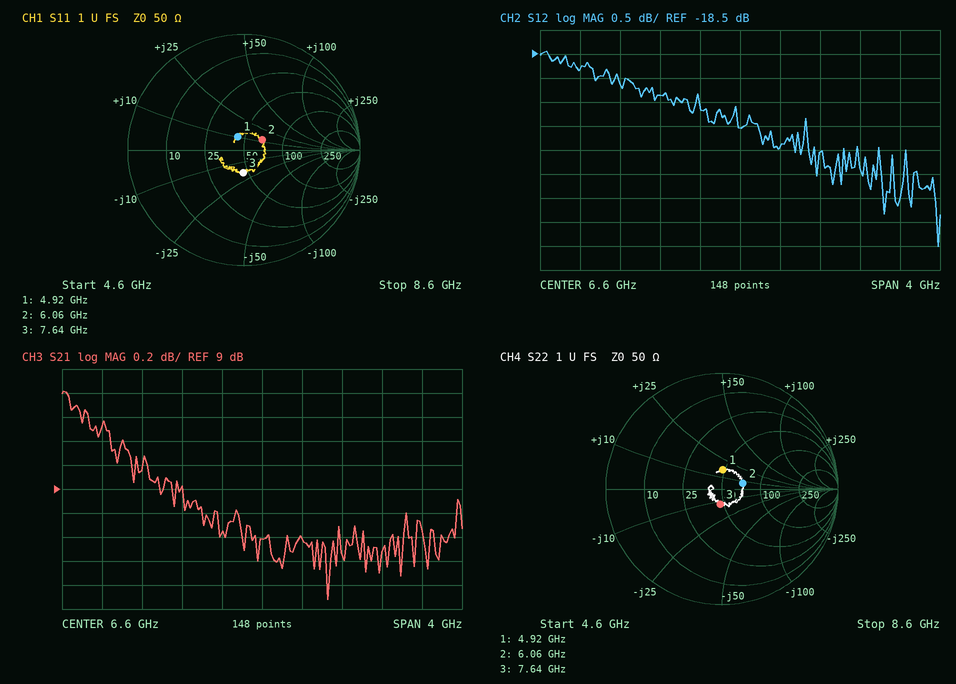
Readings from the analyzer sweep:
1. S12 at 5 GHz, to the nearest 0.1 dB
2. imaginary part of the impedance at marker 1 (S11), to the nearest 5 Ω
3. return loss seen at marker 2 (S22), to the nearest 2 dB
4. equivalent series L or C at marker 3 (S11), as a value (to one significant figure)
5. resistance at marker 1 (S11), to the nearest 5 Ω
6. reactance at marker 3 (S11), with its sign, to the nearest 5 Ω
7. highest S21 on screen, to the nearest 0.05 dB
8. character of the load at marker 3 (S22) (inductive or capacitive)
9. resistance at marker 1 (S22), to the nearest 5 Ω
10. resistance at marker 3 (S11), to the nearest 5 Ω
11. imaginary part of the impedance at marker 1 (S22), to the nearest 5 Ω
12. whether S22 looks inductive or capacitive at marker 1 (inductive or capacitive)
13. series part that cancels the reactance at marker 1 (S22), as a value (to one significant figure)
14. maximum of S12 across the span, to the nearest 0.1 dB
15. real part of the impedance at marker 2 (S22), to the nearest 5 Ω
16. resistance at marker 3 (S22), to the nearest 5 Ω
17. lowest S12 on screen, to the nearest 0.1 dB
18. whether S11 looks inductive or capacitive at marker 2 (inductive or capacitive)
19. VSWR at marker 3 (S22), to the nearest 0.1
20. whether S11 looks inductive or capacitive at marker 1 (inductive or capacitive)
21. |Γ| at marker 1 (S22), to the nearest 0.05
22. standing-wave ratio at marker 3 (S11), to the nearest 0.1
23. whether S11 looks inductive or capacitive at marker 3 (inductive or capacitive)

-18.8 dB
+10 Ω
14 dB
1 pF
45 Ω
-20 Ω
9.80 dB
capacitive
50 Ω
45 Ω
+15 Ω
inductive
2 pF
-18.4 dB
70 Ω
45 Ω
-22.5 dB
inductive
1.3
inductive
0.15
1.5
capacitive
